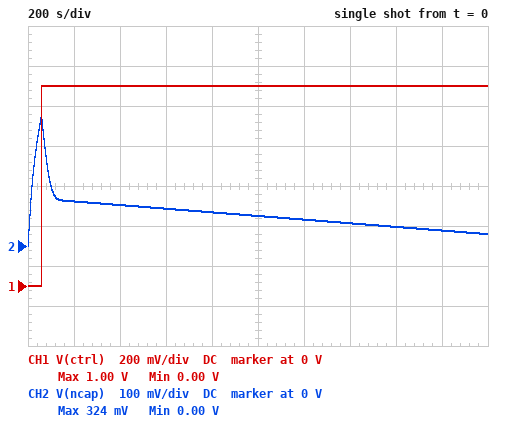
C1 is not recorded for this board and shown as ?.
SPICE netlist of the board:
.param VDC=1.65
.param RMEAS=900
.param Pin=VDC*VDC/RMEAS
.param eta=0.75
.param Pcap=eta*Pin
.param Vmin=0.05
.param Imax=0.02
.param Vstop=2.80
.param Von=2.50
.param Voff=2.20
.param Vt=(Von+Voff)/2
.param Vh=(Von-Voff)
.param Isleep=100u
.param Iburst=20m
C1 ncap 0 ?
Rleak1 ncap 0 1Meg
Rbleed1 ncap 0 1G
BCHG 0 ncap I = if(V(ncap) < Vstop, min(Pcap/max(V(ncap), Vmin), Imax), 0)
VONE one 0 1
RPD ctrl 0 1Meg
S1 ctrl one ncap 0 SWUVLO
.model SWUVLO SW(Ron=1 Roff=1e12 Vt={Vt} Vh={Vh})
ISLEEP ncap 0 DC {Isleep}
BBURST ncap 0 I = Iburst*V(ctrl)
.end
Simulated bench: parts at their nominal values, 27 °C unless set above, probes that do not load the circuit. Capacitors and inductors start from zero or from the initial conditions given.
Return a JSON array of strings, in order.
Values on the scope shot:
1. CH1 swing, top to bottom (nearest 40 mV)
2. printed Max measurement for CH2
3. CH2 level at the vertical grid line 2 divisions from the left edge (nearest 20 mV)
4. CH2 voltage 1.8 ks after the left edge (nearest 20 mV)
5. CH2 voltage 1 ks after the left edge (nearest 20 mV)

["1.00 V", "324 mV", "100 mV", "40 mV", "80 mV"]
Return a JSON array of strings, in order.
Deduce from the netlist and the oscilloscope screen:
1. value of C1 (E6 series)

["2.2 F"]
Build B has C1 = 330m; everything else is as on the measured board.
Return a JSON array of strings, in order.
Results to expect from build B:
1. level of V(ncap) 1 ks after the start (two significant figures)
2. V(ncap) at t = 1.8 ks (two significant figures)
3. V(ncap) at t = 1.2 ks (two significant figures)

["-180 mV", "-29 mV", "-240 mV"]
